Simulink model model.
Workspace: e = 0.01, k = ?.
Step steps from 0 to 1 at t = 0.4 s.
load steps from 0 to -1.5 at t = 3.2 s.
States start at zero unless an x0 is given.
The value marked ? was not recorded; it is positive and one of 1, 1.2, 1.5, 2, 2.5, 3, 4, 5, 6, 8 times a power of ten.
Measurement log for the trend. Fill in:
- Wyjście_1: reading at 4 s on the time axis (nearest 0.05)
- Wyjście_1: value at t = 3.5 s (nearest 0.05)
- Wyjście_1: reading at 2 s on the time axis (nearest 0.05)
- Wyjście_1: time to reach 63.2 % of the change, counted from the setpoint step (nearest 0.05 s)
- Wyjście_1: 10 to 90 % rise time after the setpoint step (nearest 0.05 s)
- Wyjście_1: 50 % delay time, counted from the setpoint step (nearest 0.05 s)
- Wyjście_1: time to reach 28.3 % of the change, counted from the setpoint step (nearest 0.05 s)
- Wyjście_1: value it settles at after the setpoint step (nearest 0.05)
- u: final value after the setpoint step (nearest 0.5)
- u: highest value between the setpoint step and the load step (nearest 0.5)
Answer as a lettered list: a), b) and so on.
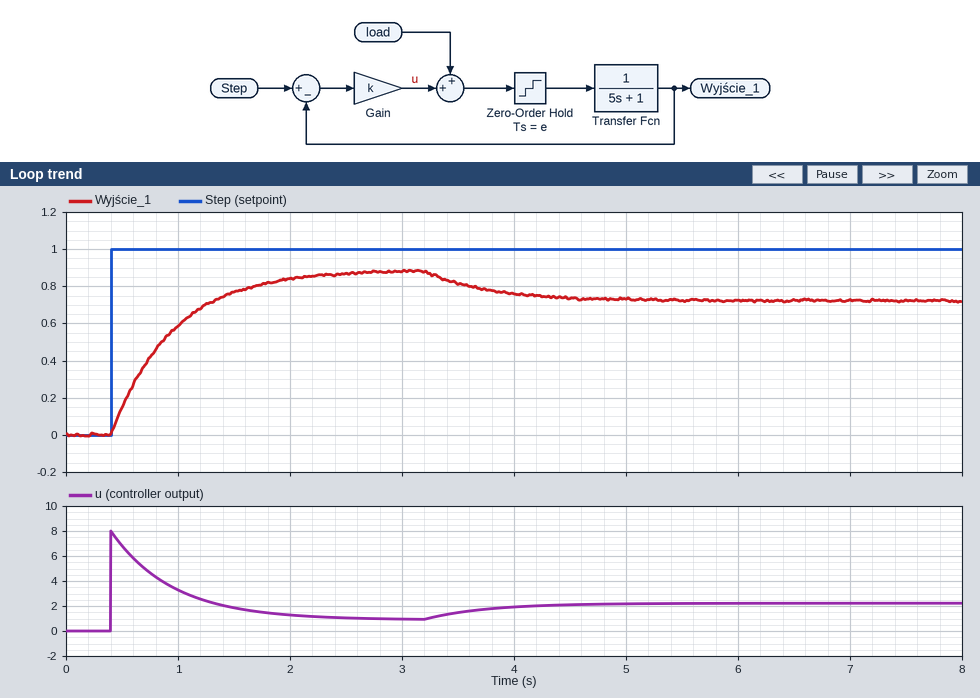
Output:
a) 0.75
b) 0.80
c) 0.85
d) 0.55 s
e) 1.20 s
f) 0.40 s
g) 0.20 s
h) 0.90
i) 1.0
j) 8.0
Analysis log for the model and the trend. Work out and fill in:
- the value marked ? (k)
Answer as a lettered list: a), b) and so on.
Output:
a) 8
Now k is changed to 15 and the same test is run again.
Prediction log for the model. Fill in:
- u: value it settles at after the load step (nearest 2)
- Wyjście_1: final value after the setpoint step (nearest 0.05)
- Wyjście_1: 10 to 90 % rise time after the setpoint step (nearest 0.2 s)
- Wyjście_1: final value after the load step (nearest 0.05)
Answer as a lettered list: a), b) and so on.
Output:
a) 2
b) 0.95
c) 0.6 s
d) 0.85
